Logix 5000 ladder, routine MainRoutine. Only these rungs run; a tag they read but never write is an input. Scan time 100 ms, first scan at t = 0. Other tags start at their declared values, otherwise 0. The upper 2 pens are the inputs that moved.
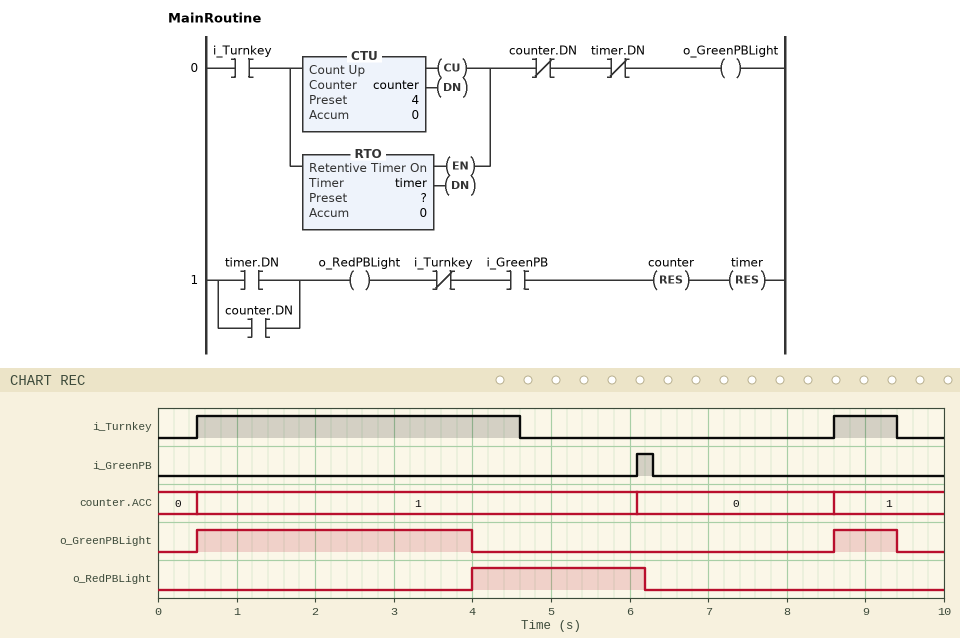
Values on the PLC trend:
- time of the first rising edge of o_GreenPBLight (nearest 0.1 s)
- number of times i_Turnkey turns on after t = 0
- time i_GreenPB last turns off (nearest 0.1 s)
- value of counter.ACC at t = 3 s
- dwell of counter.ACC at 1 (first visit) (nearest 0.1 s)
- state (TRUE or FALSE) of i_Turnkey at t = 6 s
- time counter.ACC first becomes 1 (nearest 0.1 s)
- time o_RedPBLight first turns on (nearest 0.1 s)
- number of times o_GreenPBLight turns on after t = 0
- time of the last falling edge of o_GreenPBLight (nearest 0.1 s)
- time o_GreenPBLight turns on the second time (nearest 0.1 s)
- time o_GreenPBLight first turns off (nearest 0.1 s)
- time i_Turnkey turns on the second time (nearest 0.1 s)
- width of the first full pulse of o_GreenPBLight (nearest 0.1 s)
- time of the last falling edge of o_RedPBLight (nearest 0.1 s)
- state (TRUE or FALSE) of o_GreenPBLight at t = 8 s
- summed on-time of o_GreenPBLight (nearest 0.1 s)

0.5 s
2
6.3 s
1
5.6 s
FALSE
0.5 s
4.0 s
2
9.4 s
8.6 s
4.0 s
8.6 s
3.5 s
6.2 s
FALSE
4.3 s
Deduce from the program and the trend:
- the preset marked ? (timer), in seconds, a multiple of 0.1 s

3.5 s
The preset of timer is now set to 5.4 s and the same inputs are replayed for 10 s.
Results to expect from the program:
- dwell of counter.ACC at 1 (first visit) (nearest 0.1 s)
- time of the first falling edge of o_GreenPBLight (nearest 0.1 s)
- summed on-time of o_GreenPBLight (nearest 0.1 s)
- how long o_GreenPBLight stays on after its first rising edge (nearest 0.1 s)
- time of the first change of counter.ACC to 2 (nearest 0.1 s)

8.1 s
4.6 s
4.9 s
4.1 s
8.6 s
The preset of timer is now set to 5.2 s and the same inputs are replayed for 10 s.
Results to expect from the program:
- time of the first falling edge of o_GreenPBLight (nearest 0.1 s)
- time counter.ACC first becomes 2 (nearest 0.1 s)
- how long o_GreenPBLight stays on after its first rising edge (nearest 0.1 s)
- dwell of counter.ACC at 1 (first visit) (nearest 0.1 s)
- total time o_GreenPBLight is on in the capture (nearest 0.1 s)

4.6 s
8.6 s
4.1 s
8.1 s
4.9 s
